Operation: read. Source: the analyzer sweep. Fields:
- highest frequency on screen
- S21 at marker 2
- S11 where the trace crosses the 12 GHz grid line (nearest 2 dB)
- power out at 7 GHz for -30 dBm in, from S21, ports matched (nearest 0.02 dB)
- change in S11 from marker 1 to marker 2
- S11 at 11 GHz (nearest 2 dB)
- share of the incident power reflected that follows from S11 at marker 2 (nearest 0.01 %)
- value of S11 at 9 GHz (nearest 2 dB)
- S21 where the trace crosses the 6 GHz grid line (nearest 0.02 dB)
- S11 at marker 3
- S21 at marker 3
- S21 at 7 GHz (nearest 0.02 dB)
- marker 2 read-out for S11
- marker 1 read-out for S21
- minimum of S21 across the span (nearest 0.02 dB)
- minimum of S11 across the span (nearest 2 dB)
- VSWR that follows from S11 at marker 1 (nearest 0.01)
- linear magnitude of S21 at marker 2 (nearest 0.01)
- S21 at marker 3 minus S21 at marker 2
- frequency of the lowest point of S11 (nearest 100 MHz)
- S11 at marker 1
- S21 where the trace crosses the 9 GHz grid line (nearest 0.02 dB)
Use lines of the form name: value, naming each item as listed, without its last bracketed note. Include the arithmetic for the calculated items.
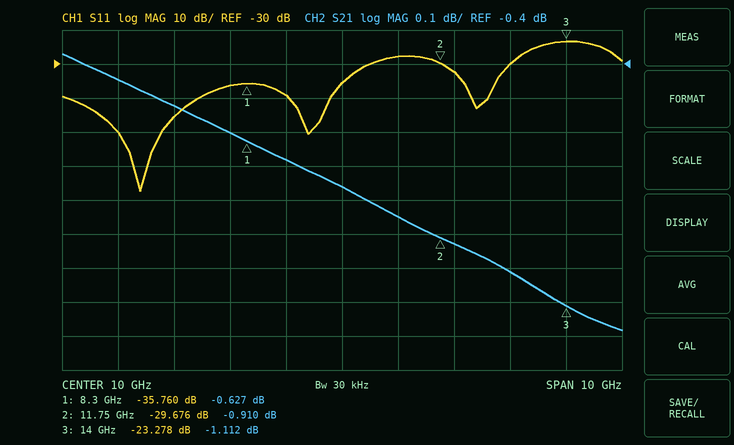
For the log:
highest frequency on screen: 15 GHz
S21 at marker 2: -0.910 dB
S11 where the trace crosses the 12 GHz grid line: -32 dB
power out at 7 GHz for -30 dBm in, from S21, ports matched: -30 dBm + (-0.52 dB) = -30.52 dBm
change in S11 from marker 1 to marker 2: -29.676 − (-35.76) = 6.084 dB
S11 at 11 GHz: -28 dB
share of the incident power reflected that follows from S11 at marker 2: 10^(-29.676/10) ≈ 0.11 %
value of S11 at 9 GHz: -40 dB
S21 where the trace crosses the 6 GHz grid line: -0.44 dB
S11 at marker 3: -23.278 dB
S21 at marker 3: -1.112 dB
S21 at 7 GHz: -0.52 dB
marker 2 read-out for S11: -29.676 dB
marker 1 read-out for S21: -0.627 dB
minimum of S21 across the span: -1.18 dB
minimum of S11 across the span: -68 dB
VSWR that follows from S11 at marker 1: (1 + 0.0163)/(1 − 0.0163) ≈ 1.03
linear magnitude of S21 at marker 2: 10^(-0.91/20) ≈ 0.90
S21 at marker 3 minus S21 at marker 2: -1.112 − (-0.91) = -0.202 dB
frequency of the lowest point of S11: 6.4 GHz
S11 at marker 1: -35.760 dB
S21 where the trace crosses the 9 GHz grid line: -0.68 dB
